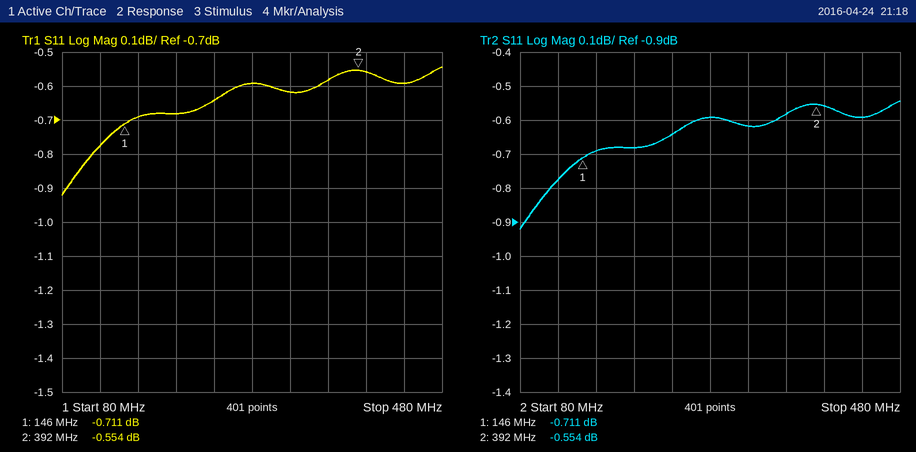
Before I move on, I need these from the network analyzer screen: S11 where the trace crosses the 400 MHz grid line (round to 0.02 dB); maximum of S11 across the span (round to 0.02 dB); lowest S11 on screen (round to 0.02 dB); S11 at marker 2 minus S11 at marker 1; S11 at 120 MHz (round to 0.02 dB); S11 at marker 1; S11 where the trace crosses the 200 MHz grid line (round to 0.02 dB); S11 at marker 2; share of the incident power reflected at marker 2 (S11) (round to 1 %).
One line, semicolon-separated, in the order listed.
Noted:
-0.56 dB; -0.54 dB; -0.92 dB; 0.157 dB; -0.78 dB; -0.711 dB; -0.68 dB; -0.554 dB; 88 %
